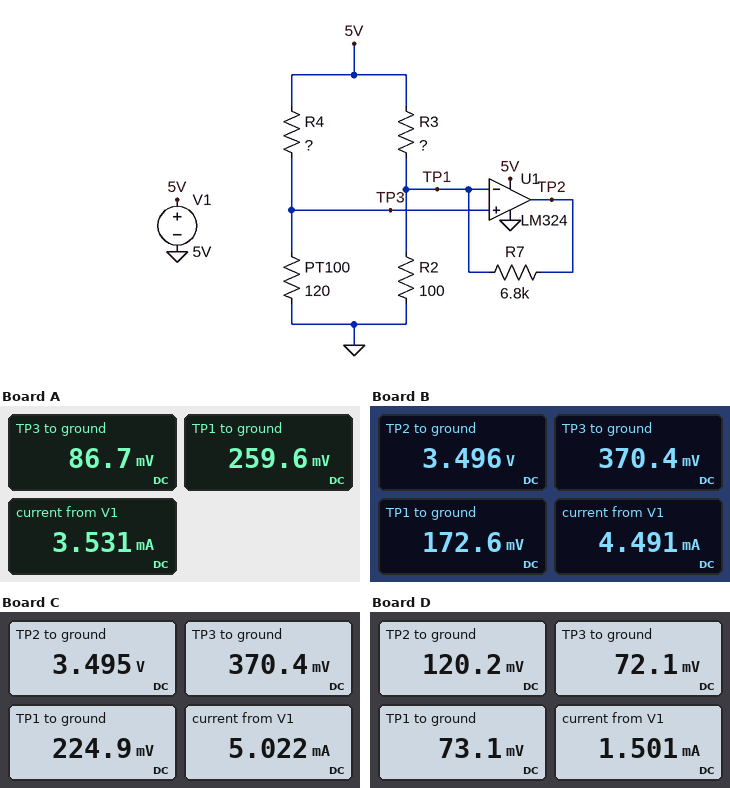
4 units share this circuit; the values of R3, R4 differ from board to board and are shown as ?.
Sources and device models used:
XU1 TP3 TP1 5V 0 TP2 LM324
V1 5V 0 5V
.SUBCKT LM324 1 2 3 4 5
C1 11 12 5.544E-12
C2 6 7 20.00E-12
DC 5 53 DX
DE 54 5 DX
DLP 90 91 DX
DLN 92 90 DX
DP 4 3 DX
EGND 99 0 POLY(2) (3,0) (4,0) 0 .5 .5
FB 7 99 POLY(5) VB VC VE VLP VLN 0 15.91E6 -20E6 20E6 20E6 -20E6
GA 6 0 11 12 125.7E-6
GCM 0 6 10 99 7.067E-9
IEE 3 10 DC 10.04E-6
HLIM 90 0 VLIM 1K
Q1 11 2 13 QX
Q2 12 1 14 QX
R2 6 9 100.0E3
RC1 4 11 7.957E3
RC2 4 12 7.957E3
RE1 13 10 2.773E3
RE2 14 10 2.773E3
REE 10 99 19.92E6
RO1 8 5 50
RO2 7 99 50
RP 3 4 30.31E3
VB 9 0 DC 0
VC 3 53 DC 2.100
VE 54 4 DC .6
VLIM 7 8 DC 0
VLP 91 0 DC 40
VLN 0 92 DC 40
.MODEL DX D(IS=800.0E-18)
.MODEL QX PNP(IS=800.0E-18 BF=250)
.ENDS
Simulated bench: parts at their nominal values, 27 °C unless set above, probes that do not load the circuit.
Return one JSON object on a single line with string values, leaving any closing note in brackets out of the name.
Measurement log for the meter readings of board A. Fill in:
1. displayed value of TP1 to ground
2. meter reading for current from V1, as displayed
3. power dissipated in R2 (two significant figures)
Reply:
{"displayed value of TP1 to ground": "259.6 mV", "meter reading for current from V1, as displayed": "3.531 mA", "power dissipated in R2": "670 µW"}
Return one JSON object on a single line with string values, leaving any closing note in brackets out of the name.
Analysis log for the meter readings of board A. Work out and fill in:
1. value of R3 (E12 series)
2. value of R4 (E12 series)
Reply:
{"value of R3": "1.8 kΩ", "value of R4": "6.8 kΩ"}
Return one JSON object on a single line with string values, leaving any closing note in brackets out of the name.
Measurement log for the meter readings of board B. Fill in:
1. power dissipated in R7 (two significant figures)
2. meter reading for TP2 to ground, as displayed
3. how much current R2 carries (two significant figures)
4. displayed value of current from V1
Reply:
{"power dissipated in R7": "1.6 mW", "meter reading for TP2 to ground, as displayed": "3.496 V", "how much current R2 carries": "1.7 mA", "displayed value of current from V1": "4.491 mA"}
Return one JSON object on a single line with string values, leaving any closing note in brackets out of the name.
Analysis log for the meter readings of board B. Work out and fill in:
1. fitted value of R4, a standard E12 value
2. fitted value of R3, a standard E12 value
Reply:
{"fitted value of R4, a standard E12 value": "1.5 kΩ", "fitted value of R3, a standard E12 value": "3.9 kΩ"}
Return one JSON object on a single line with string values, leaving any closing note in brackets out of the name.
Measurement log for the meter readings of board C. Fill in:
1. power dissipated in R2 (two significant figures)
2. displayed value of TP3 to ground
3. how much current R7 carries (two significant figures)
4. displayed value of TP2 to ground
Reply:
{"power dissipated in R2": "510 µW", "displayed value of TP3 to ground": "370.4 mV", "how much current R7 carries": "480 µA", "displayed value of TP2 to ground": "3.495 V"}
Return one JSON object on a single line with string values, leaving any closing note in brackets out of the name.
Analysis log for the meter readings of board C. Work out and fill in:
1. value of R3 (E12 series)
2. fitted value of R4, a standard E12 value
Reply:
{"value of R3": "2.7 kΩ", "fitted value of R4, a standard E12 value": "1.5 kΩ"}
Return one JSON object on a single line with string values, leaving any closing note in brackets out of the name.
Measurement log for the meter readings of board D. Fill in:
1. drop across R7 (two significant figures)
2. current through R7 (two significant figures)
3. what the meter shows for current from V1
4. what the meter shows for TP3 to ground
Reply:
{"drop across R7": "47 mV", "current through R7": "6.9 µA", "what the meter shows for current from V1": "1.501 mA", "what the meter shows for TP3 to ground": "72.1 mV"}
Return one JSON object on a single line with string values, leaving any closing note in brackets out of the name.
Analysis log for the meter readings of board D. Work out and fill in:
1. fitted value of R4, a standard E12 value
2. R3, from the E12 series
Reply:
{"fitted value of R4, a standard E12 value": "8.2 kΩ", "R3, from the E12 series": "6.8 kΩ"}
